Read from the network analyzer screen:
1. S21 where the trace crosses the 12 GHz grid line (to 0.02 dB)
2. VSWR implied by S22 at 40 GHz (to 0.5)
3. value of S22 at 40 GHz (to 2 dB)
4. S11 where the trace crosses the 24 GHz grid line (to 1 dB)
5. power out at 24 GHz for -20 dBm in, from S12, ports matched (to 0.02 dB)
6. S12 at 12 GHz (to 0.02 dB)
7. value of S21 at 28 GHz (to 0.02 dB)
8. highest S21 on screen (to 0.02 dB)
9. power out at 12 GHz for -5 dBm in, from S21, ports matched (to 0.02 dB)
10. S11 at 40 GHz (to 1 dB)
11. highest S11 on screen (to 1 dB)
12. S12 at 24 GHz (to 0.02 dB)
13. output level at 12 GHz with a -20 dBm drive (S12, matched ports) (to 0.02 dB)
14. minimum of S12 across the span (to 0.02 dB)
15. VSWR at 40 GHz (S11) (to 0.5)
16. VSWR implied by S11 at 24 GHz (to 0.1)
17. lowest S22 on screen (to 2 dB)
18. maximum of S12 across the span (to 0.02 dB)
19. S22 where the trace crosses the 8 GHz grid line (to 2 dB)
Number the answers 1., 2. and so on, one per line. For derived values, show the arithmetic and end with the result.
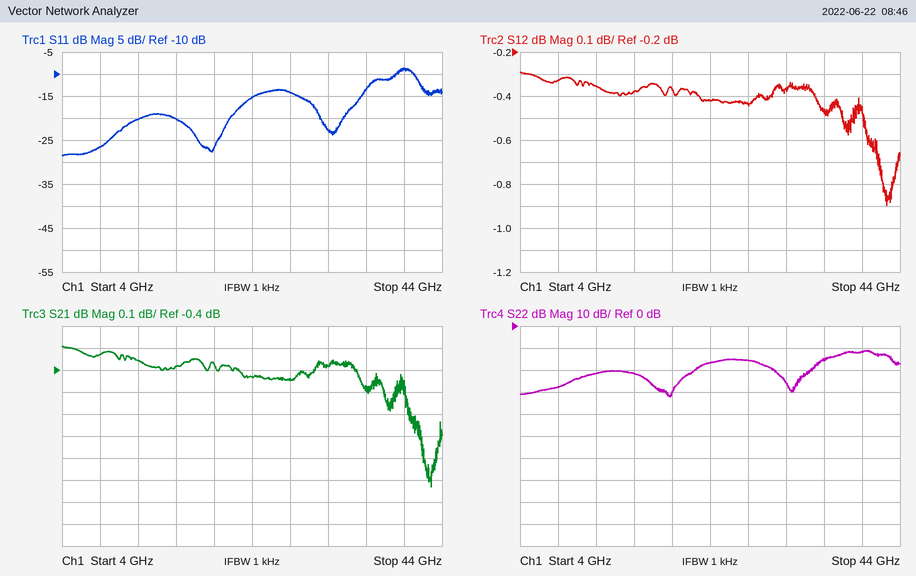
1. -0.36 dB
2. |Γ| = 10^(-12/20) = 0.2512; VSWR = (1 + 0.2512)/(1 − 0.2512) ≈ 1.67, so 1.5 to the nearest 0.5
3. -12 dB
4. -15 dB
5. -20 dBm + (-0.42 dB) = -20.42 dBm
6. -0.36 dB
7. -0.44 dB
8. -0.30 dB
9. -5 dBm + (-0.36 dB) = -5.36 dBm
10. -9 dB
11. -9 dB
12. -0.42 dB
13. -20 dBm + (-0.36 dB) = -20.36 dBm
14. -0.90 dB
15. |Γ| = 10^(-9/20) = 0.3548; VSWR = (1 + 0.3548)/(1 − 0.3548) ≈ 2.10, so 2.0 to the nearest 0.5
16. |Γ| = 10^(-15/20) = 0.1778; VSWR = (1 + 0.1778)/(1 − 0.1778) ≈ 1.4
17. -32 dB
18. -0.30 dB
19. -28 dB
